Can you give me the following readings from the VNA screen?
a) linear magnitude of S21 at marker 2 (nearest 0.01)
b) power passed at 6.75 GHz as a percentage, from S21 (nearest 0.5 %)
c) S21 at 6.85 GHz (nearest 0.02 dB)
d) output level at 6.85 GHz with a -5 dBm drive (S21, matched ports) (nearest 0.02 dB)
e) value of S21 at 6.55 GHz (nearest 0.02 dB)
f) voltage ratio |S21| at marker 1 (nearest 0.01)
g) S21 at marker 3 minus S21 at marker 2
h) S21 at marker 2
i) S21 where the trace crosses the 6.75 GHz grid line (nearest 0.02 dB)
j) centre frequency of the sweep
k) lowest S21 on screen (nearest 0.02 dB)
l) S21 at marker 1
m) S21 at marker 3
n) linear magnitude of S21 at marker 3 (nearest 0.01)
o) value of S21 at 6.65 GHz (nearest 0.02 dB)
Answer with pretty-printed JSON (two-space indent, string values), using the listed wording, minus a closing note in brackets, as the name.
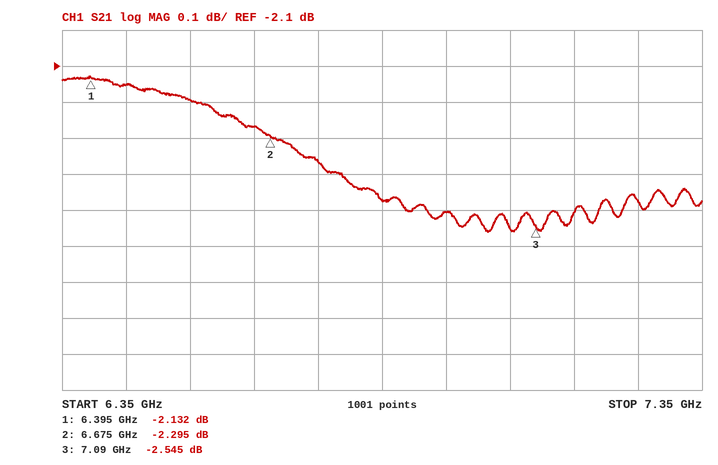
{
  "linear magnitude of S21 at marker 2": "0.77",
  "power passed at 6.75 GHz as a percentage, from S21": "58.0 %",
  "S21 at 6.85 GHz": "-2.48 dB",
  "output level at 6.85 GHz with a -5 dBm drive (S21, matched ports)": "-7.48 dBm",
  "value of S21 at 6.55 GHz": "-2.20 dB",
  "voltage ratio |S21| at marker 1": "0.78",
  "S21 at marker 3 minus S21 at marker 2": "-0.250 dB",
  "S21 at marker 2": "-2.295 dB",
  "S21 where the trace crosses the 6.75 GHz grid line": "-2.36 dB",
  "centre frequency of the sweep": "6.85 GHz",
  "lowest S21 on screen": "-2.56 dB",
  "S21 at marker 1": "-2.132 dB",
  "S21 at marker 3": "-2.545 dB",
  "linear magnitude of S21 at marker 3": "0.75",
  "value of S21 at 6.65 GHz": "-2.26 dB"
}
